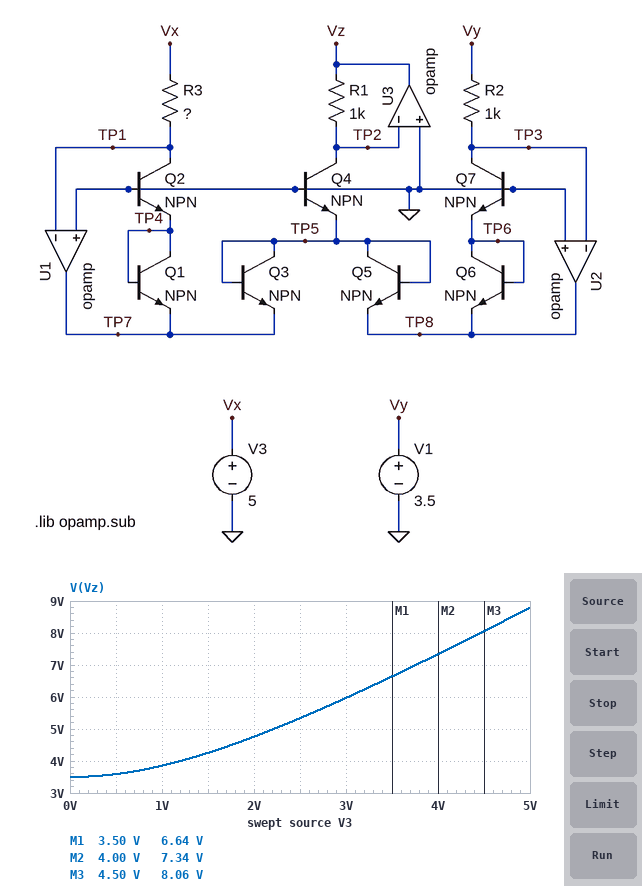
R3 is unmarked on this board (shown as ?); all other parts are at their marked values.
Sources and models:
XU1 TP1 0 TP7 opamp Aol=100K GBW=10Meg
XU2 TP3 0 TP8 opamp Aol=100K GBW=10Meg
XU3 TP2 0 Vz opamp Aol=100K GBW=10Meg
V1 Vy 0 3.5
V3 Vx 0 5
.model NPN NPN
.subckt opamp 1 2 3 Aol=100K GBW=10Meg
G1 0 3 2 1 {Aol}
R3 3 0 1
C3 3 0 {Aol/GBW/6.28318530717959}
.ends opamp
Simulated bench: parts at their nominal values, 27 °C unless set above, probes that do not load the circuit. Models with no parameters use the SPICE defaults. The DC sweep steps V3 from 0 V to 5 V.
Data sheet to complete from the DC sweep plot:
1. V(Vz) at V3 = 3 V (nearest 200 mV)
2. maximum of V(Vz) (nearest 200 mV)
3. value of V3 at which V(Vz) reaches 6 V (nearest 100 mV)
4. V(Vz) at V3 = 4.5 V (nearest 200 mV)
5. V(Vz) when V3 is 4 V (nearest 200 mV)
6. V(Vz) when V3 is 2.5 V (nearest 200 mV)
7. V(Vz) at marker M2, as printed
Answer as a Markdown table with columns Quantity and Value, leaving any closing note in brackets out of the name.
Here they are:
| Quantity | Value |
|---|---|
| V(Vz) at V3 = 3 V | 6.0 V |
| maximum of V(Vz) | 8.8 V |
| value of V3 at which V(Vz) reaches 6 V | 3.0 V |
| V(Vz) at V3 = 4.5 V | 8.0 V |
| V(Vz) when V3 is 4 V | 7.4 V |
| V(Vz) when V3 is 2.5 V | 5.4 V |
| V(Vz) at marker M2, as printed | 7.34 V |
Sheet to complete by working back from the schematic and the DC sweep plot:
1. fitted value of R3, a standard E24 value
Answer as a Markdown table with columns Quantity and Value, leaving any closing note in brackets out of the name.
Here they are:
| Quantity | Value |
|---|---|
| fitted value of R3, a standard E24 value | 620 Ω |
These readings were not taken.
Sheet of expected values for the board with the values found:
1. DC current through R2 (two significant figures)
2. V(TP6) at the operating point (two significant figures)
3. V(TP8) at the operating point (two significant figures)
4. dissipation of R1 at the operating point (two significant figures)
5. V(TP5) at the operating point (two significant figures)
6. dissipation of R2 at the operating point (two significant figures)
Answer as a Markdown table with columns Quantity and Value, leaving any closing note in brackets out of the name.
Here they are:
| Quantity | Value |
|---|---|
| DC current through R2 | 3.5 mA |
| V(TP6) at the operating point | -810 mV |
| V(TP8) at the operating point | -1.6 V |
| dissipation of R1 at the operating point | 77 mW |
| V(TP5) at the operating point | -830 mV |
| dissipation of R2 at the operating point | 12 mW |
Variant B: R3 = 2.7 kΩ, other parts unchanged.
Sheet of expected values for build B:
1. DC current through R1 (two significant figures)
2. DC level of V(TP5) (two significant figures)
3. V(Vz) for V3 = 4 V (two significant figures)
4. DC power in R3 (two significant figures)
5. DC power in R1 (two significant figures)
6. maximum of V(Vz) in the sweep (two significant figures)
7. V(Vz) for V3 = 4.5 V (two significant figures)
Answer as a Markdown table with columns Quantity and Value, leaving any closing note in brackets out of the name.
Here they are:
| Quantity | Value |
|---|---|
| DC current through R1 | 4.0 mA |
| DC level of V(TP5) | -810 mV |
| V(Vz) for V3 = 4 V | 3.8 V |
| DC power in R3 | 9.3 mW |
| DC power in R1 | 16 mW |
| maximum of V(Vz) in the sweep | 4.0 V |
| V(Vz) for V3 = 4.5 V | 3.9 V |
